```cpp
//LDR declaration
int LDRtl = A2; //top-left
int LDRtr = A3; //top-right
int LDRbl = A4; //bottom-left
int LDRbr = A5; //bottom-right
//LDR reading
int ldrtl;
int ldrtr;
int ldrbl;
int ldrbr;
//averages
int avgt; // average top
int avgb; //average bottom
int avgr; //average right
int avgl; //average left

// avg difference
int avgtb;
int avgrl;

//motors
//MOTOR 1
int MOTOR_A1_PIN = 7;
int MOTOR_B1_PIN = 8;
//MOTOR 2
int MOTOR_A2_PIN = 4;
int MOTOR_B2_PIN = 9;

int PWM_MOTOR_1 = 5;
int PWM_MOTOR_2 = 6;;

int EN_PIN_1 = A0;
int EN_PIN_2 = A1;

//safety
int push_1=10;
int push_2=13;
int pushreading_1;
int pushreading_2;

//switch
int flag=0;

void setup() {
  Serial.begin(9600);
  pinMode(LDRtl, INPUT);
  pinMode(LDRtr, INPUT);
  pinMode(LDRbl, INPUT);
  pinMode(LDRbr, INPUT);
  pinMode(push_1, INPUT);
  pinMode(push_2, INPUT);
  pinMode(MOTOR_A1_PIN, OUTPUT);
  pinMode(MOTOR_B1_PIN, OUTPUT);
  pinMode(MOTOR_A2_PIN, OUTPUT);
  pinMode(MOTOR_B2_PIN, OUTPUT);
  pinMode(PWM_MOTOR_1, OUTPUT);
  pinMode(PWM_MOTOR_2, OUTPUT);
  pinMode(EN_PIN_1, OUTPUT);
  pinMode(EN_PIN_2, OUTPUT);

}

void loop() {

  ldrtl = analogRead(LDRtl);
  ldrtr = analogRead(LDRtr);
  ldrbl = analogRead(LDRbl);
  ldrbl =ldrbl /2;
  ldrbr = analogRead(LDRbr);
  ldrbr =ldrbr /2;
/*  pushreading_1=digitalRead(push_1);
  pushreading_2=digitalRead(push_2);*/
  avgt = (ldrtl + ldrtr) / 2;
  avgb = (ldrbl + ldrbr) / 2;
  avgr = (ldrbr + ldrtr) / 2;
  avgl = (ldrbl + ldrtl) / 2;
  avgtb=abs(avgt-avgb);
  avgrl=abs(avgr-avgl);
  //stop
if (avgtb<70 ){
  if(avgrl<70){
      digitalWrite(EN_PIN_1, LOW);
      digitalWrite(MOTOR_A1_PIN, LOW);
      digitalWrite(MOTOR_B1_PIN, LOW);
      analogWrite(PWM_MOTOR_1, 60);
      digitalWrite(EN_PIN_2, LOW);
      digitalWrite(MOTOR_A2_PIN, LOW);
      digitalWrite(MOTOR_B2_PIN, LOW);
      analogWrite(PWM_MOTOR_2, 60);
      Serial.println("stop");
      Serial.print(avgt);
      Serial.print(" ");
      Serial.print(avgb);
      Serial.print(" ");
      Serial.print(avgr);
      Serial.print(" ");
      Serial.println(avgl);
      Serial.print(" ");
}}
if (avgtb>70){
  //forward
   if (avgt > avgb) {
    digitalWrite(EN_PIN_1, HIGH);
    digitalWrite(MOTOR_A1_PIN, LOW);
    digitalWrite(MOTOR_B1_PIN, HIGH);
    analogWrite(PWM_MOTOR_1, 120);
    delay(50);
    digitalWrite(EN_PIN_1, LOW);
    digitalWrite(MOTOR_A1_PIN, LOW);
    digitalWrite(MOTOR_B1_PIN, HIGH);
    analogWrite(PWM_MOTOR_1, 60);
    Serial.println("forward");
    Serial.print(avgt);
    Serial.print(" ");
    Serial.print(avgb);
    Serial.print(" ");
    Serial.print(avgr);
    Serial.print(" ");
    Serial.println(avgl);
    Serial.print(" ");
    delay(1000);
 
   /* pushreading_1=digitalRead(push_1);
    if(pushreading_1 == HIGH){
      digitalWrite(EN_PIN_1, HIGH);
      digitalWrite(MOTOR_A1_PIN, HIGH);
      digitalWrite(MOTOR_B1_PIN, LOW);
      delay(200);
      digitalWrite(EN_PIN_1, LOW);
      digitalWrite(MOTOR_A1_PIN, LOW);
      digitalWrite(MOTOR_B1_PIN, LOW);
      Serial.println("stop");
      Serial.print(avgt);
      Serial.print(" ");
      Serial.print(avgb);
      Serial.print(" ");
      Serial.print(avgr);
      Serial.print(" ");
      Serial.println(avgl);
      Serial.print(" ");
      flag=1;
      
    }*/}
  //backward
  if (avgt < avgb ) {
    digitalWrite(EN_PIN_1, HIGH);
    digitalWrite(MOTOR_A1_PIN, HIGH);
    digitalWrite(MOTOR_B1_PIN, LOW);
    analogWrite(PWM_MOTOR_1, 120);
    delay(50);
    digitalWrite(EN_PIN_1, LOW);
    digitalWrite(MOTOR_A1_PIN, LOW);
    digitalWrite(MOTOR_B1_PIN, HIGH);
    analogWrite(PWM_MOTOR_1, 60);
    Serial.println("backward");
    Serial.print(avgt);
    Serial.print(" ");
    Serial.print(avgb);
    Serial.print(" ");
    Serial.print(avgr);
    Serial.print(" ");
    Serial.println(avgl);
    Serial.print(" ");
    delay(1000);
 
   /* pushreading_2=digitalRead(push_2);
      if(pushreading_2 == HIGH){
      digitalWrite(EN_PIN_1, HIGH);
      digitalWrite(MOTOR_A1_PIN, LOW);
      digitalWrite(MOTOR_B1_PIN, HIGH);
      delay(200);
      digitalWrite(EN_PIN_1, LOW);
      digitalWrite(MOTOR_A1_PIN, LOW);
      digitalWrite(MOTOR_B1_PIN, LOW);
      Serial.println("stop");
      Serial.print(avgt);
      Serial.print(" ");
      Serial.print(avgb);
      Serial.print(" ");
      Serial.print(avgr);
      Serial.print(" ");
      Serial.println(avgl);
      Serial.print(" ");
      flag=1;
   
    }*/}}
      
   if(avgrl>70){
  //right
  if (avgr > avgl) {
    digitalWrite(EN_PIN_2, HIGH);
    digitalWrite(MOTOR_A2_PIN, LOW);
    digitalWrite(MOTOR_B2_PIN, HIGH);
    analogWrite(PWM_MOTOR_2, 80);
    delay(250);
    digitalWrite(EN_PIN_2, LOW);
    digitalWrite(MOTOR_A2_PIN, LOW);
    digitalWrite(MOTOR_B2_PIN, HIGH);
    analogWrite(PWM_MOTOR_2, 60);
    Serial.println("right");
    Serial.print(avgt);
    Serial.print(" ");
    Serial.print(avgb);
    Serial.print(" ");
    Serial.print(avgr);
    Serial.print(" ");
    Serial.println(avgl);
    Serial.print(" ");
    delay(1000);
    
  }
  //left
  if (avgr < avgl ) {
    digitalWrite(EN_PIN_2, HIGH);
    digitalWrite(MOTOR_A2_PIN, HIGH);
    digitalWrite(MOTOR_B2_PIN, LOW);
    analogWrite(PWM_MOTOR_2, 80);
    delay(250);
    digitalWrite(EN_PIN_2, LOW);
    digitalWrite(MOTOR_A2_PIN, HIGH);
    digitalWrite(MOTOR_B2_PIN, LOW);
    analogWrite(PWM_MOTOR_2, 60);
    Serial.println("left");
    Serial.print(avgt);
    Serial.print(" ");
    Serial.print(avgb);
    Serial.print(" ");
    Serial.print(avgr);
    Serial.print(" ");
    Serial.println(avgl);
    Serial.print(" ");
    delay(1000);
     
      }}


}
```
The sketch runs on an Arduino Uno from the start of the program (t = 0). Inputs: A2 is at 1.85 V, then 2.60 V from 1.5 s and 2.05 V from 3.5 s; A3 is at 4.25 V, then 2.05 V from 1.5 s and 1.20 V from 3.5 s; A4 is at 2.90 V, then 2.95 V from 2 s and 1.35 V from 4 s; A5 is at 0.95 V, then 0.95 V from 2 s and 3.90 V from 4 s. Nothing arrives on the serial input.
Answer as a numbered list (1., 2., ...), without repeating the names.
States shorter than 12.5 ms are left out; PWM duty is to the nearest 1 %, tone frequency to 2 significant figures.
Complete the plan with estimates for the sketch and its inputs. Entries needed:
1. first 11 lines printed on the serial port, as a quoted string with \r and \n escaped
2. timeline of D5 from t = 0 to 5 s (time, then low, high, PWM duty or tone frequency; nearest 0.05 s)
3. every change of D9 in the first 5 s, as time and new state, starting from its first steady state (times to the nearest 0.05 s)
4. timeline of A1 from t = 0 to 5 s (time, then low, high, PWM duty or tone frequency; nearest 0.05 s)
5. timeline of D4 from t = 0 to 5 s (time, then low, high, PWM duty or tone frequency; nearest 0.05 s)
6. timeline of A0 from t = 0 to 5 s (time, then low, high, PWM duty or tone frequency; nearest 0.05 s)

1. "forward\r\n624 196 483 337\r\n right\r\n624 196 483 337\r\n forward\r\n475 199 258 417\r\n left\r\n475 199 258 417\r\n stop\r\n332 268 322 278\r\n stop\r\n"
2. 0 s PWM 47 %; 0.05 s PWM 24 %; 2.3 s PWM 47 %; 2.35 s PWM 24 %
3. 0 s low; 1.05 s high; 3.35 s low
4. 0 s low; 1.05 s high; 1.3 s low; 3.35 s high; 3.6 s low
5. 0 s low; 3.35 s high; 4.6 s low
6. 0 s high; 0.05 s low; 2.3 s high; 2.35 s low
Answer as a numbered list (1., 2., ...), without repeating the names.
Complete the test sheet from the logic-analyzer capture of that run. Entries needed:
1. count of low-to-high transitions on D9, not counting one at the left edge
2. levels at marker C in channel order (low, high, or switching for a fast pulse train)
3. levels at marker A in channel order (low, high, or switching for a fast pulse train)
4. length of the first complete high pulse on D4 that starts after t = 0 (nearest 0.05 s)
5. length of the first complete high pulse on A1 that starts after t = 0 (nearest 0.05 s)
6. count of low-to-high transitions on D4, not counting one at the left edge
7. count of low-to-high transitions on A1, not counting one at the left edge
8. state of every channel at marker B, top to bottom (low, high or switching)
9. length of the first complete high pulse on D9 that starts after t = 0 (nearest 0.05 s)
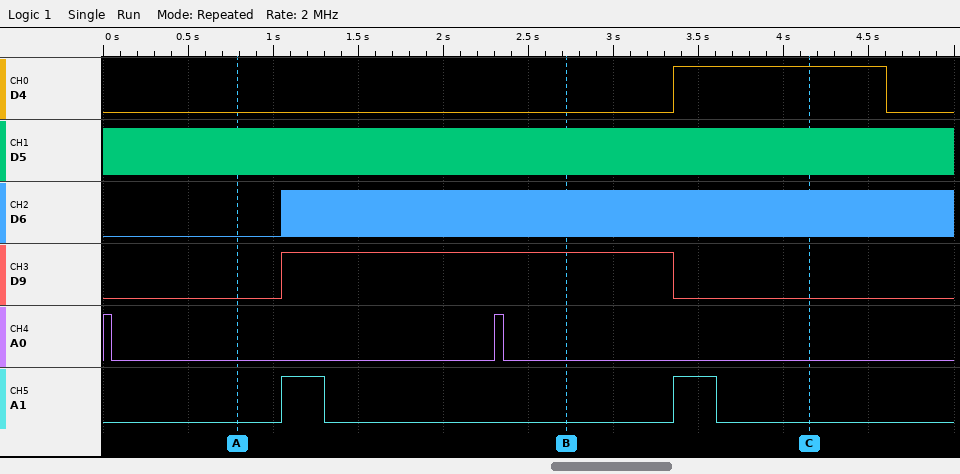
1. 1
2. D4 high, D5 switching, D6 switching, D9 low, A0 low, A1 low
3. D4 low, D5 switching, D6 low, D9 low, A0 low, A1 low
4. 1.25 s
5. 0.25 s
6. 1
7. 2
8. D4 low, D5 switching, D6 switching, D9 high, A0 low, A1 low
9. 2.30 s
